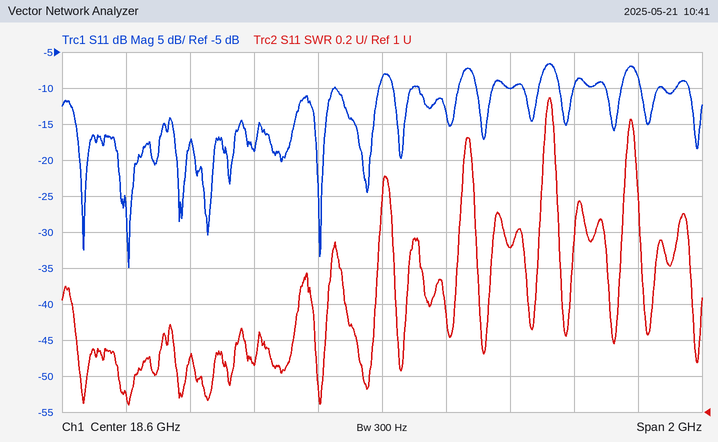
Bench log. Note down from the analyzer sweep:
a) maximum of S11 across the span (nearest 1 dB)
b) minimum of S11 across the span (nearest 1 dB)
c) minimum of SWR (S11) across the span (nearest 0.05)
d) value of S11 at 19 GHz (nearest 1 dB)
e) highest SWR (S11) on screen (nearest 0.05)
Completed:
-7 dB
-35 dB
1.05
-10 dB
2.75
